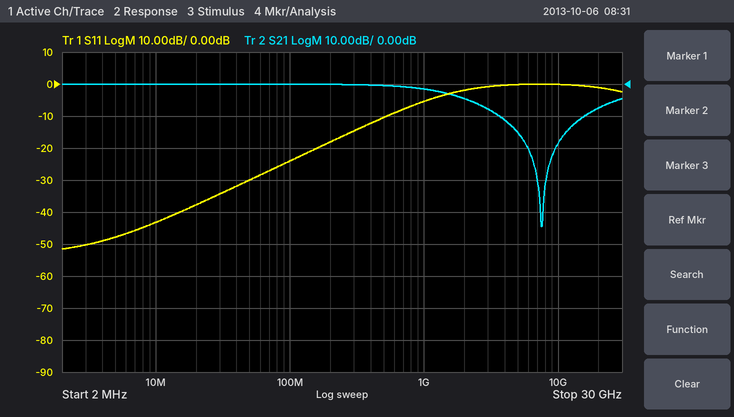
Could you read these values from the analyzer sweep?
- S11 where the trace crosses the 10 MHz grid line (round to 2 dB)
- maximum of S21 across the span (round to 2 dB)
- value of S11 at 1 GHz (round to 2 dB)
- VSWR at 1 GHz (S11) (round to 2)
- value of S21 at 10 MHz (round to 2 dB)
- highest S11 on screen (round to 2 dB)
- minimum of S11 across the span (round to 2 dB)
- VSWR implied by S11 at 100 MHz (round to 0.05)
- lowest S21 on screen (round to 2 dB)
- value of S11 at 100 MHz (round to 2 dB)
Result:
-44 dB
0 dB
-6 dB
4
0 dB
0 dB
-52 dB
1.15
-44 dB
-24 dB
